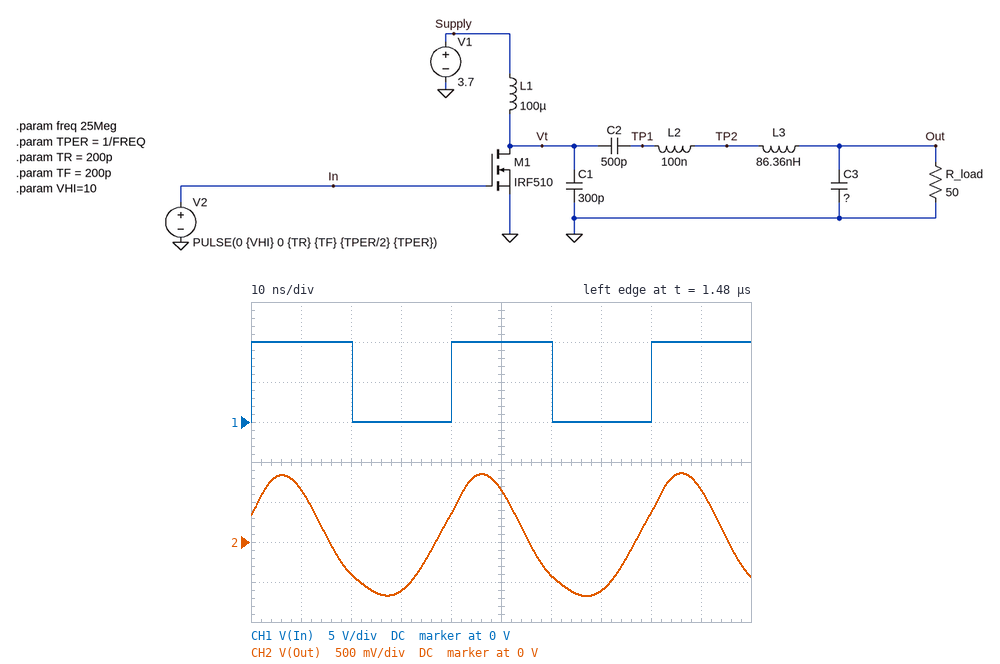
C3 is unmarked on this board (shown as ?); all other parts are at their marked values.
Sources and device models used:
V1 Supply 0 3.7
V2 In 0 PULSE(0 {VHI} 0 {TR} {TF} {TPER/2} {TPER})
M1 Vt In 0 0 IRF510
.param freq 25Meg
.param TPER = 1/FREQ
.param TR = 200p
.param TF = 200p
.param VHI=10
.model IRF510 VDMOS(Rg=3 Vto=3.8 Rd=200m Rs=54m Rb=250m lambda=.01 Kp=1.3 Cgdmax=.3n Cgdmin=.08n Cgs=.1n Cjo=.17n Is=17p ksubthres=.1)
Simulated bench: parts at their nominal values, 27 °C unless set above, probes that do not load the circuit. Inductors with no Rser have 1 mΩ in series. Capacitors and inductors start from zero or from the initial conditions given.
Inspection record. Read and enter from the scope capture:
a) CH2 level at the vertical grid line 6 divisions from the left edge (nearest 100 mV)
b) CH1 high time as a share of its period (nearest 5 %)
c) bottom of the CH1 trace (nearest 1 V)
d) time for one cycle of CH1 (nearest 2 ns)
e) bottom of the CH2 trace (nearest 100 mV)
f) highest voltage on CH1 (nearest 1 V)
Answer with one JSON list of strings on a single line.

["-400 mV", "50 %", "0 V", "40 ns", "-700 mV", "10 V"]
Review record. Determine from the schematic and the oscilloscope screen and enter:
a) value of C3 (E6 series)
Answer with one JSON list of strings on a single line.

["220 pF"]
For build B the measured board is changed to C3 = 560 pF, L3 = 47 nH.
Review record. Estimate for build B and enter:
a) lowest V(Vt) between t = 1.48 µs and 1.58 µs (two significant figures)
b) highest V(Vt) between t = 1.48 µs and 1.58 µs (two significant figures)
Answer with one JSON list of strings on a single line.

["-760 mV", "1.8 V"]
